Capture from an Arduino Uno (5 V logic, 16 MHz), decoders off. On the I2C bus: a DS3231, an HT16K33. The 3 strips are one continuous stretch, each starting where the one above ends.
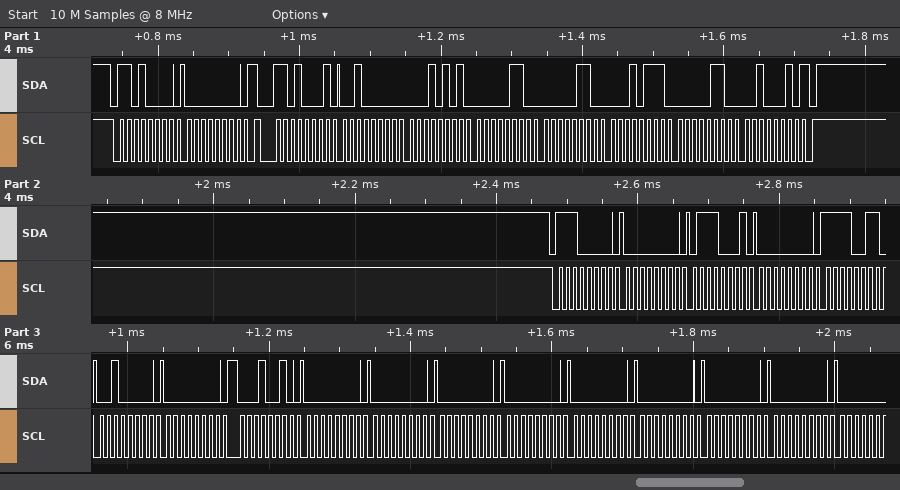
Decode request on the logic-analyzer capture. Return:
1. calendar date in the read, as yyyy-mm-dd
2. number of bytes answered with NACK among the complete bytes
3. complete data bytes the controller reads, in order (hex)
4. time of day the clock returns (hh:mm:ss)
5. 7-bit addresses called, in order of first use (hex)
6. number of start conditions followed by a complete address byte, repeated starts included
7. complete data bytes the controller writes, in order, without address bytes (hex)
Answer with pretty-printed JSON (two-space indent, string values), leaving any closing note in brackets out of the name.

{
  "calendar date in the read, as yyyy-mm-dd": "2022-06-17",
  "number of bytes answered with NACK among the complete bytes": "1",
  "complete data bytes the controller reads, in order": "20 15 06 06 17 06 22",
  "time of day the clock returns": "06:15:20",
  "7-bit addresses called, in order of first use": "0x68 0x70",
  "number of start conditions followed by a complete address byte, repeated starts included": "3",
  "complete data bytes the controller writes, in order, without address bytes": "00 00 71 00 F3 20 00 12 00 00 00 00 00 00 00 00"
}
